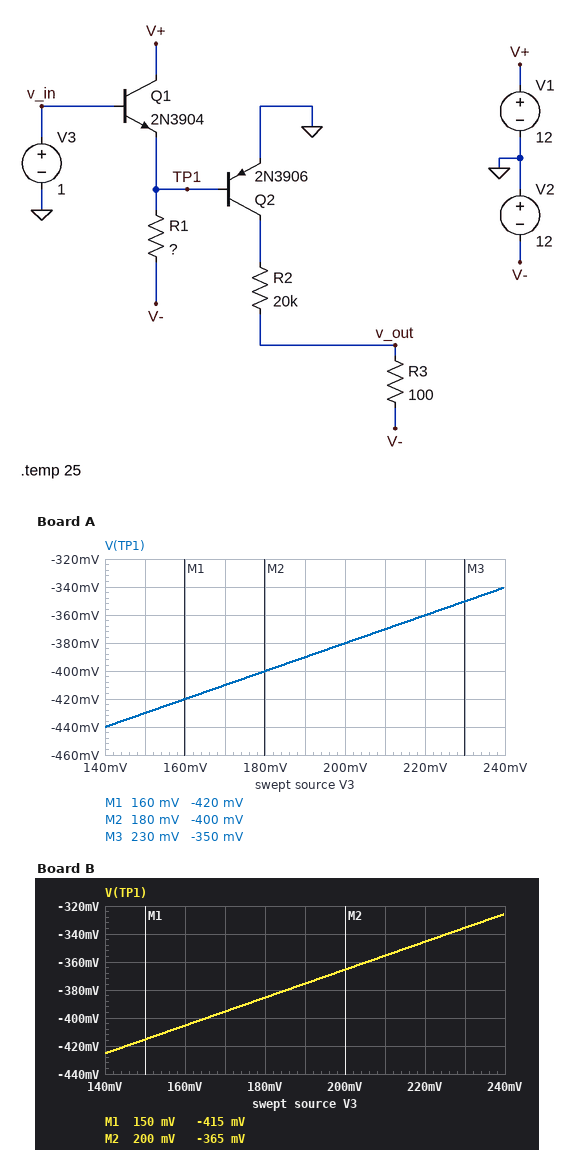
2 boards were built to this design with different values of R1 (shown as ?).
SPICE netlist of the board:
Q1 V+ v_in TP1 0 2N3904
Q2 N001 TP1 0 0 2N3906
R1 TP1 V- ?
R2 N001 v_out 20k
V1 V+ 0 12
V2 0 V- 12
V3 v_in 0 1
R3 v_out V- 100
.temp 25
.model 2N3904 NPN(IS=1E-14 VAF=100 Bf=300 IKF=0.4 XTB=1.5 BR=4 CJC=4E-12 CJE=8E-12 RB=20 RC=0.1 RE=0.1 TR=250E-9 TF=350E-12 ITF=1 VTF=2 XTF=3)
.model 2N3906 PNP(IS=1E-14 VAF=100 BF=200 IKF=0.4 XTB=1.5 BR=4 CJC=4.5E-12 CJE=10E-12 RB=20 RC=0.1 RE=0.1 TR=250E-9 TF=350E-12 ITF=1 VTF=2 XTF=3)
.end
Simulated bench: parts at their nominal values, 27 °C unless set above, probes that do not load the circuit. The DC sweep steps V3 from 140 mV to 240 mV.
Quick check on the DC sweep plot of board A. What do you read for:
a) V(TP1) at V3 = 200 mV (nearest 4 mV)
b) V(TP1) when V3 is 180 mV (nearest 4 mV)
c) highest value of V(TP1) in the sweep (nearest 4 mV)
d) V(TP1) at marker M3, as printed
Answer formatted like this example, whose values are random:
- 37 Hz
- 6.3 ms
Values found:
- -380 mV
- -400 mV
- -340 mV
- -350 mV
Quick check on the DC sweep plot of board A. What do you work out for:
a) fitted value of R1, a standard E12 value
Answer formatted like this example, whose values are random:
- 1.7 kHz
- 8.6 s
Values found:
- 220 kΩ
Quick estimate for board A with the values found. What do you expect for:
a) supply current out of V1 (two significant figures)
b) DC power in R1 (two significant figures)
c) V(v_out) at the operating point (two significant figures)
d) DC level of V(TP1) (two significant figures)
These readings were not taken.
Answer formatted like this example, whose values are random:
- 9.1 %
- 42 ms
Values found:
- 56 µA
- 700 µW
- -12 V
- 420 mV
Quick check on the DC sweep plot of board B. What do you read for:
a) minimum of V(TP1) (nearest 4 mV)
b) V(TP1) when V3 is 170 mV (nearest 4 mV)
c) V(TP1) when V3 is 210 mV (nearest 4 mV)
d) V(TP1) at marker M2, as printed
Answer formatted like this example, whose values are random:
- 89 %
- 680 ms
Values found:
- -424 mV
- -396 mV
- -356 mV
- -365 mV
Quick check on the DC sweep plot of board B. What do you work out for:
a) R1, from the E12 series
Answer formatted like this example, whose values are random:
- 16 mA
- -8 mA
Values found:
- 390 kΩ
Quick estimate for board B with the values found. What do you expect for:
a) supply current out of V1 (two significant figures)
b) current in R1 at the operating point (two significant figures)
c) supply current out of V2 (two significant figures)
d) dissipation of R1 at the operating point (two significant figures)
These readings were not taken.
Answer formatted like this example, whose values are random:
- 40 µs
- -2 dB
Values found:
- 32 µA
- 32 µA
- 32 µA
- 400 µW
